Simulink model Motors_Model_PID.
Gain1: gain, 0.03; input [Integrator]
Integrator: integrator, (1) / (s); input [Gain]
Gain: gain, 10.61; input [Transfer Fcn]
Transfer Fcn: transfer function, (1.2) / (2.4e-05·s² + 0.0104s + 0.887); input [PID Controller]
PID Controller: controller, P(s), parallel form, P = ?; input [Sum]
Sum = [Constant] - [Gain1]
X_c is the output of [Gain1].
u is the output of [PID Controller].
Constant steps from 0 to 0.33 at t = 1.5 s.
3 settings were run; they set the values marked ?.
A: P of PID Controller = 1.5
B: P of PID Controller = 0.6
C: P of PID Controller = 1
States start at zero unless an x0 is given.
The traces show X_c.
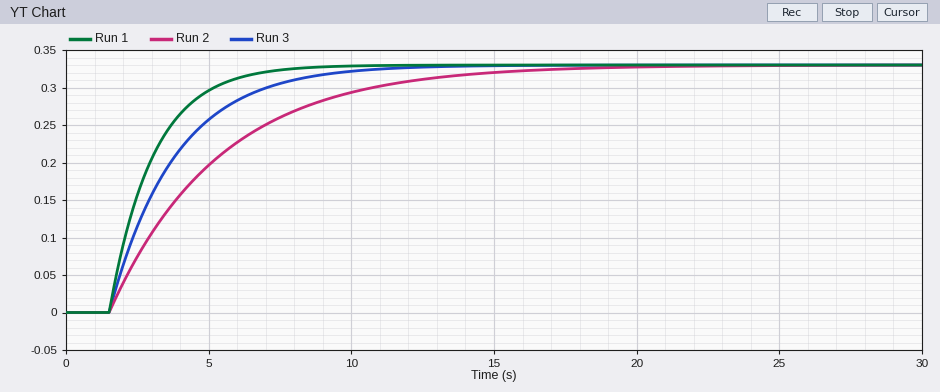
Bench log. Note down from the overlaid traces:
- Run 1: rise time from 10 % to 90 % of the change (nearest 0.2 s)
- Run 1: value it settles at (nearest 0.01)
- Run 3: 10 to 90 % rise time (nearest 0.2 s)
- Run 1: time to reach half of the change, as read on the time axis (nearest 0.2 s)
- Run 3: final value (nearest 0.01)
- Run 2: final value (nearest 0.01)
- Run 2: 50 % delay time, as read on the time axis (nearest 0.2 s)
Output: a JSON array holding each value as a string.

["3.4 s", "0.33", "5.0 s", "2.6 s", "0.33", "0.33", "4.2 s"]
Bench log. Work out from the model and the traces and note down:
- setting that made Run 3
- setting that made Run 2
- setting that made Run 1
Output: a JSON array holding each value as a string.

["C", "B", "A"]
